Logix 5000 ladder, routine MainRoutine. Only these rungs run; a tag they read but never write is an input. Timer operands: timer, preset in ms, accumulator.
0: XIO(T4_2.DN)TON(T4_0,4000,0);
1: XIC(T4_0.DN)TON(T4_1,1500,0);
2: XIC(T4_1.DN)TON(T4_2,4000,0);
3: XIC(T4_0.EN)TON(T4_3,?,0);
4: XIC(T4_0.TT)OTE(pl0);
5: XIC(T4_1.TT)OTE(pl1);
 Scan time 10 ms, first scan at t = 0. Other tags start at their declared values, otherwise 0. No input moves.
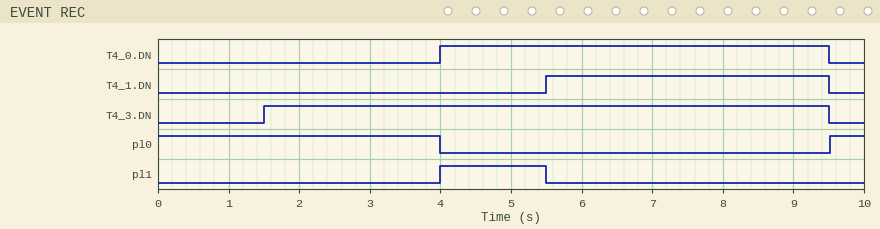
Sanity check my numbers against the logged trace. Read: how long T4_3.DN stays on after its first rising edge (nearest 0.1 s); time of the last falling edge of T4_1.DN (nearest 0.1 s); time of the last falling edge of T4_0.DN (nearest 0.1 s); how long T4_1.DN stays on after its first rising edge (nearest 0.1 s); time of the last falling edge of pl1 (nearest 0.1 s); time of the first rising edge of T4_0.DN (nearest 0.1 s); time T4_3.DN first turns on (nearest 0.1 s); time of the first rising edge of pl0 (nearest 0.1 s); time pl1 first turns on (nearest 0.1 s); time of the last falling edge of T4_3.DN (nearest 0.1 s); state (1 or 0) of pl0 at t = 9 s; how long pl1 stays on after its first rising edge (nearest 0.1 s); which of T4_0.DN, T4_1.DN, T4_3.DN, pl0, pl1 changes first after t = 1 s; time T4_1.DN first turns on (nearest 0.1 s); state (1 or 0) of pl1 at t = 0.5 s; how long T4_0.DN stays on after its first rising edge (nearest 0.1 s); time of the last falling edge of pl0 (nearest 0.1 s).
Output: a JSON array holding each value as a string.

["8.0 s", "9.5 s", "9.5 s", "4.0 s", "5.5 s", "4.0 s", "1.5 s", "9.5 s", "4.0 s", "9.5 s", "0", "1.5 s", "T4_3.DN", "5.5 s", "0", "5.5 s", "4.0 s"]
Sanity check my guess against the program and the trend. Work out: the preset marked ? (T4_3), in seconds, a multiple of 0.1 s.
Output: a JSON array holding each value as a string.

["1.5 s"]
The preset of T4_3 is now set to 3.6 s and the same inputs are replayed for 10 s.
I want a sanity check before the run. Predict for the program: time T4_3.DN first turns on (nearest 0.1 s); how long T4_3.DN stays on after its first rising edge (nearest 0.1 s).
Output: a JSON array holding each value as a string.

["3.6 s", "5.9 s"]
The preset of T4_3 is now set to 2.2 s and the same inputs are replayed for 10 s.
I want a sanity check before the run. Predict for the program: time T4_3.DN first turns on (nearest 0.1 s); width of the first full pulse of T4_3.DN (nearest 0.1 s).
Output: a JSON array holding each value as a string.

["2.2 s", "7.3 s"]
